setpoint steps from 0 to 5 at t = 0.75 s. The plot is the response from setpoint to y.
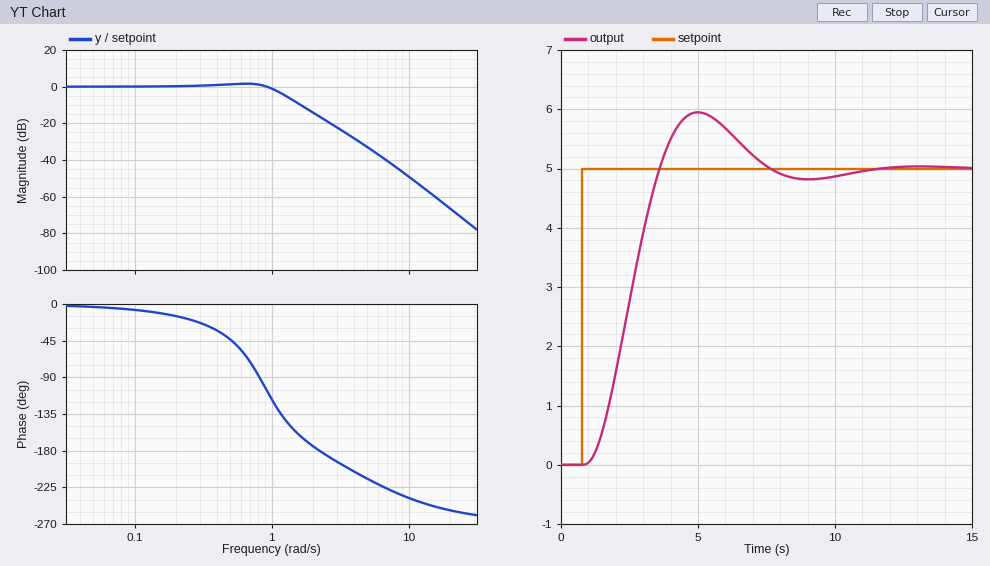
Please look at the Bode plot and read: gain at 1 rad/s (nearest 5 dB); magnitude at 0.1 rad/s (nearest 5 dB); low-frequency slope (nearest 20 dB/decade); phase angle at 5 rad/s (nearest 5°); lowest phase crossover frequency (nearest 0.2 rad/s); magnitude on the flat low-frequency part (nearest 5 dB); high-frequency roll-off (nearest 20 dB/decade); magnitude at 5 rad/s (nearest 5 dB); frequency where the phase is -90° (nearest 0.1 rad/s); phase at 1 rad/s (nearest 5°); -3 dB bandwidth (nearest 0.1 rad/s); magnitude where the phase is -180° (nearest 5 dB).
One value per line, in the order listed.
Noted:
0 dB
0 dB
0 dB/decade
-215°
2.2 rad/s
0 dB
-60 dB/decade
-35 dB
0.8 rad/s
-115°
1.1 rad/s
-15 dB
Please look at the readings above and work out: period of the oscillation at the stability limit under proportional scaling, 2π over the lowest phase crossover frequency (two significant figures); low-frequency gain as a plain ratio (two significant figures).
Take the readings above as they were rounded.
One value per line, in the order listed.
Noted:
2.9 s
1.0
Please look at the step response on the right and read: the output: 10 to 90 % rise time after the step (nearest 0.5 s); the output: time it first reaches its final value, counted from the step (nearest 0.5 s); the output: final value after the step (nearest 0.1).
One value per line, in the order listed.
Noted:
2.0 s
3.0 s
5.0
